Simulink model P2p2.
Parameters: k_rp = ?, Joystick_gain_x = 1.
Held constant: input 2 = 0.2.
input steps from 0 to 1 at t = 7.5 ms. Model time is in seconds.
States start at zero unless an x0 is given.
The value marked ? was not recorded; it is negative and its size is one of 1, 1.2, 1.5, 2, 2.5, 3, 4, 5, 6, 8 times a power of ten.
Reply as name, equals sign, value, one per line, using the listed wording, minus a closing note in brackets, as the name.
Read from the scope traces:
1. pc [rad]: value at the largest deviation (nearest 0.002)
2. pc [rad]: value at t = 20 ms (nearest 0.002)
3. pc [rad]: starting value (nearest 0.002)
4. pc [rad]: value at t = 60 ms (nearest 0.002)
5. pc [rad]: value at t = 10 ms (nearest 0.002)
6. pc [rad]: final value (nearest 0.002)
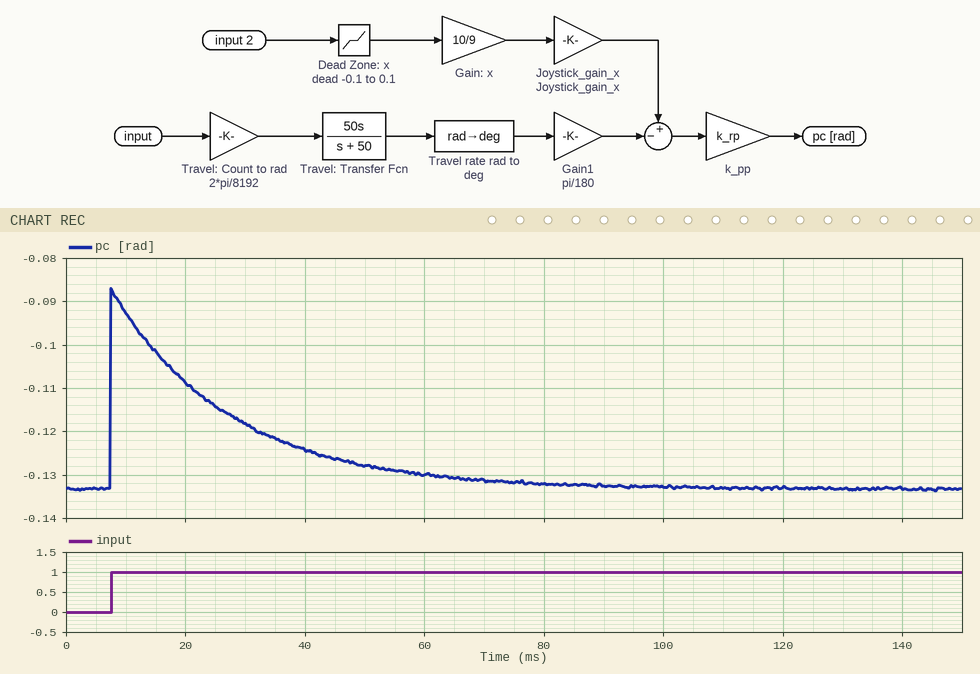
pc [rad]: value at the largest deviation = -0.088
pc [rad]: value at t = 20 ms = -0.108
pc [rad]: starting value = -0.134
pc [rad]: value at t = 60 ms = -0.130
pc [rad]: value at t = 10 ms = -0.092
pc [rad]: final value = -0.134
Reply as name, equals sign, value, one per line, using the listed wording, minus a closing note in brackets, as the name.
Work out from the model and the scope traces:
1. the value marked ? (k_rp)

the value marked ? = -1.2
